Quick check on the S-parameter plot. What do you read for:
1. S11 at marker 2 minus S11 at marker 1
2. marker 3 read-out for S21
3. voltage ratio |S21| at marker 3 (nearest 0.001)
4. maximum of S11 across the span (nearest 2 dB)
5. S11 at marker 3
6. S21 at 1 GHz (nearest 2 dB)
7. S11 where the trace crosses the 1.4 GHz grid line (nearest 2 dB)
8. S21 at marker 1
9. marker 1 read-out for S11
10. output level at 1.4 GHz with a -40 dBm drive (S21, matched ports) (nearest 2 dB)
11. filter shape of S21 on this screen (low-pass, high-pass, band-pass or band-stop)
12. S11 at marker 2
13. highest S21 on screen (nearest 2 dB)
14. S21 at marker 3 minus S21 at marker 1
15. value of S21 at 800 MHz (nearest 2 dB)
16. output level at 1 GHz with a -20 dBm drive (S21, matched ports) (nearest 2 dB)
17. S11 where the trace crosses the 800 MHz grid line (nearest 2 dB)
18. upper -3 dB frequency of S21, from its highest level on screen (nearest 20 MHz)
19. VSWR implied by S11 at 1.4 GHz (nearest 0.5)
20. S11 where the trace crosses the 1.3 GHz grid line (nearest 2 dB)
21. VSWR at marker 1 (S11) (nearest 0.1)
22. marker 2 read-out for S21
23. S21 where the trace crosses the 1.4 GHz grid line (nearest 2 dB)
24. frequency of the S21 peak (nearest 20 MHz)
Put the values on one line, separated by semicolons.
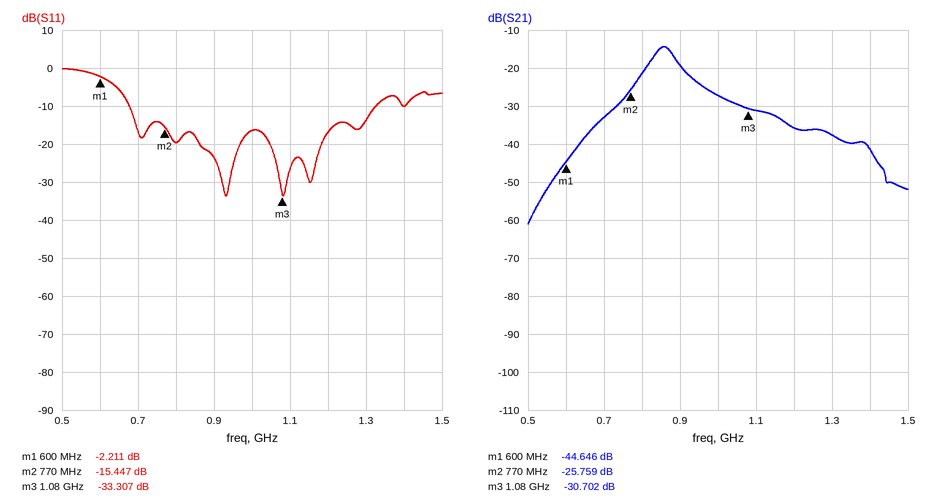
-13.236 dB; -30.702 dB; 0.029; 0 dB; -33.307 dB; -28 dB; -10 dB; -44.646 dB; -2.211 dB; -82 dBm; band-pass; -15.447 dB; -14 dB; 13.944 dB; -22 dB; -48 dBm; -20 dB; 880 MHz; 2.0; -14 dB; 7.9; -25.759 dB; -42 dB; 860 MHz
